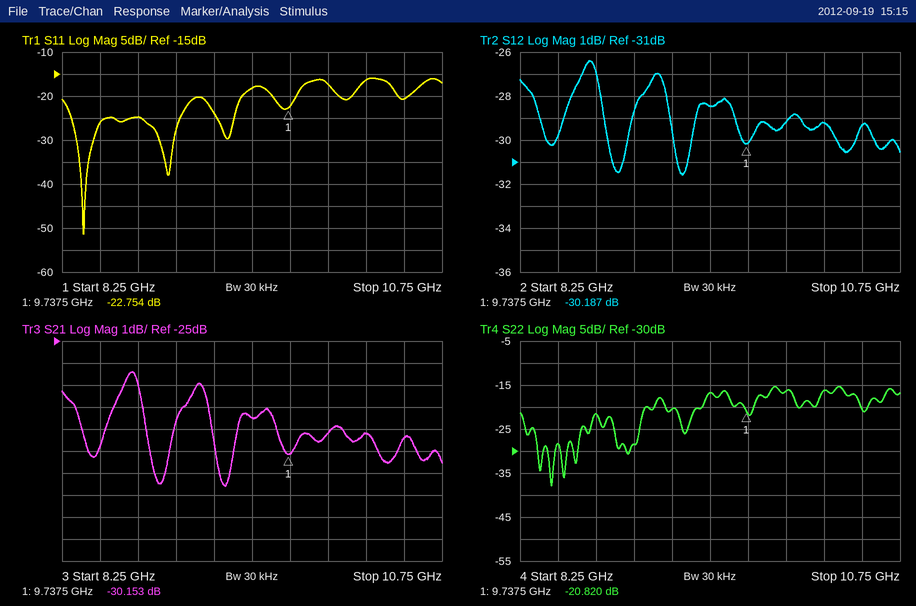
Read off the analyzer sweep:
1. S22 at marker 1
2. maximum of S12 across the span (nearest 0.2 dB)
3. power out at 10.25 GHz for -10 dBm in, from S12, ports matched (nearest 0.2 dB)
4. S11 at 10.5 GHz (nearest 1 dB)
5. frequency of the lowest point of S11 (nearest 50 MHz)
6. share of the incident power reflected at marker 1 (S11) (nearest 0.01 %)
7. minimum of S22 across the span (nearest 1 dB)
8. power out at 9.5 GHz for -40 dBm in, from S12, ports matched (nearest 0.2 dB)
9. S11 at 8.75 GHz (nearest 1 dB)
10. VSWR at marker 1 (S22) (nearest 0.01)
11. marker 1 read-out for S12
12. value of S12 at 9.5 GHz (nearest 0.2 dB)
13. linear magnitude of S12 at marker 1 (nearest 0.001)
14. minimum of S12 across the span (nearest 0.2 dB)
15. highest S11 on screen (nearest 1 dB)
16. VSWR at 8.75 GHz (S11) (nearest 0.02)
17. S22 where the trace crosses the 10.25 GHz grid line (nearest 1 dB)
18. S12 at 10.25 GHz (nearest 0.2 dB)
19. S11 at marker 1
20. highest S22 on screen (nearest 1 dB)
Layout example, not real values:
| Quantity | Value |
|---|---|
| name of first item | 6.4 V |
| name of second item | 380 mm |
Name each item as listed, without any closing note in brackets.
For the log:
| Quantity | Value |
|---|---|
| S22 at marker 1 | -20.820 dB |
| maximum of S12 across the span | -26.4 dB |
| power out at 10.25 GHz for -10 dBm in, from S12, ports matched | -39.2 dBm |
| S11 at 10.5 GHz | -21 dB |
| frequency of the lowest point of S11 | 8.40 GHz |
| share of the incident power reflected at marker 1 (S11) | 0.53 % |
| minimum of S22 across the span | -38 dB |
| power out at 9.5 GHz for -40 dBm in, from S12, ports matched | -68.4 dBm |
| S11 at 8.75 GHz | -25 dB |
| VSWR at marker 1 (S22) | 1.20 |
| marker 1 read-out for S12 | -30.187 dB |
| value of S12 at 9.5 GHz | -28.4 dB |
| linear magnitude of S12 at marker 1 | 0.031 |
| minimum of S12 across the span | -31.6 dB |
| highest S11 on screen | -16 dB |
| VSWR at 8.75 GHz (S11) | 1.12 |
| S22 where the trace crosses the 10.25 GHz grid line | -16 dB |
| S12 at 10.25 GHz | -29.2 dB |
| S11 at marker 1 | -22.754 dB |
| highest S22 on screen | -15 dB |
